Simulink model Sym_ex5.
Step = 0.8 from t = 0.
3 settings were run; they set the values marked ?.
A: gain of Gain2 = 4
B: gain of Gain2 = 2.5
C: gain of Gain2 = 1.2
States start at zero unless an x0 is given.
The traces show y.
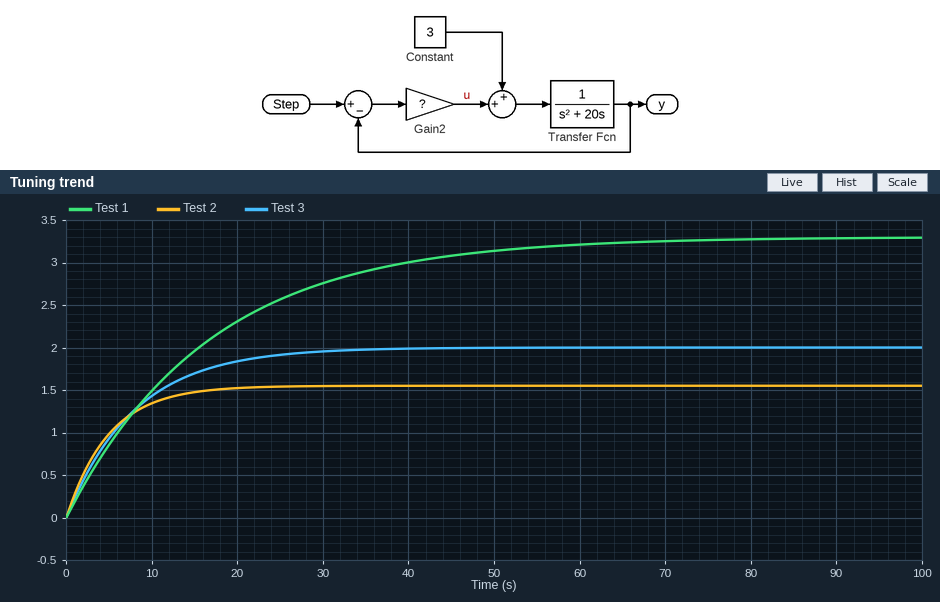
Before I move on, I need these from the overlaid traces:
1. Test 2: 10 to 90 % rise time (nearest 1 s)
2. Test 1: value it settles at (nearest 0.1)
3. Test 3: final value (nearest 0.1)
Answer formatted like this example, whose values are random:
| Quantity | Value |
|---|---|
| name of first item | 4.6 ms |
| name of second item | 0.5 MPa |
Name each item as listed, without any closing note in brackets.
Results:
| Quantity | Value |
|---|---|
| Test 2: 10 to 90 % rise time | 11 s |
| Test 1: value it settles at | 3.3 |
| Test 3: final value | 2.0 |
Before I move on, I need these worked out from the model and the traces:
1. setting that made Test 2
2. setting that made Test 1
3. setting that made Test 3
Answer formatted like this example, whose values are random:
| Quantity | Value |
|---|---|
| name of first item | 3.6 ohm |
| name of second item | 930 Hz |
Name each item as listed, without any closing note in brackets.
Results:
| Quantity | Value |
|---|---|
| setting that made Test 2 | A |
| setting that made Test 1 | C |
| setting that made Test 3 | B |
